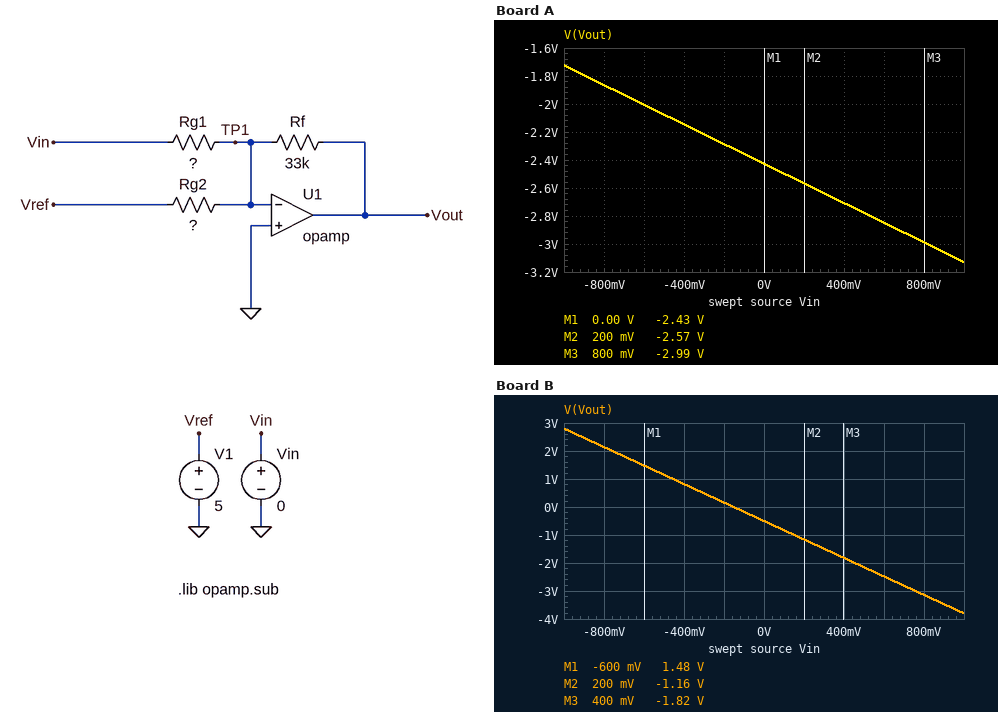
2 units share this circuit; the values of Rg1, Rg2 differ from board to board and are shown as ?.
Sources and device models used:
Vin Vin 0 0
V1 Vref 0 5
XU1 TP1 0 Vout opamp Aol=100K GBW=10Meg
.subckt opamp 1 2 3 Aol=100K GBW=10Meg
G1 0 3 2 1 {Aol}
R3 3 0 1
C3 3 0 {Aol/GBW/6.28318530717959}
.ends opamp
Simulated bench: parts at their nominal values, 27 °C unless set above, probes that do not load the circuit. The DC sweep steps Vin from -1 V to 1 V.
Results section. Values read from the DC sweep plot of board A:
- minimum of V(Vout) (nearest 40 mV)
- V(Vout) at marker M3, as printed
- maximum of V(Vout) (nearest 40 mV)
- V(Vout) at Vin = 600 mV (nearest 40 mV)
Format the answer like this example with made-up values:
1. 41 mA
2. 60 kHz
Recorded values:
1. -3.12 V
2. -2.99 V
3. -1.72 V
4. -2.84 V
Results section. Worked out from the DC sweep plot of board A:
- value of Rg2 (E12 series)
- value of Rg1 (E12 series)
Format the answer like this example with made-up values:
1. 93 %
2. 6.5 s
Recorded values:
1. 68 kΩ
2. 47 kΩ
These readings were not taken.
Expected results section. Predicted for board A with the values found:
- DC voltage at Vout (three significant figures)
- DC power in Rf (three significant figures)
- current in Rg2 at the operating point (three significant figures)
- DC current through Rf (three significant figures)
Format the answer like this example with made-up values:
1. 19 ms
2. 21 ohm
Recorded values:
1. -2.43 V
2. 178 µW
3. 73.5 µA
4. 73.5 µA
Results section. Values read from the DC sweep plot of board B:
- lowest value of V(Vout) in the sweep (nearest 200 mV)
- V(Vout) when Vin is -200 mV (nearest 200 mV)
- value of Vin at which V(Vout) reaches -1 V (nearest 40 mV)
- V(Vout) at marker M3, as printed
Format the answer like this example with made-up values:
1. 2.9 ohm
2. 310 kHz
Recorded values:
1. -3.8 V
2. 200 mV
3. 160 mV
4. -1.82 V
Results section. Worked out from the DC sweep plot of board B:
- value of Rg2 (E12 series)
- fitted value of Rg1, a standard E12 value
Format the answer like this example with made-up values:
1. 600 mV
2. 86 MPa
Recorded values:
1. 330 kΩ
2. 10 kΩ
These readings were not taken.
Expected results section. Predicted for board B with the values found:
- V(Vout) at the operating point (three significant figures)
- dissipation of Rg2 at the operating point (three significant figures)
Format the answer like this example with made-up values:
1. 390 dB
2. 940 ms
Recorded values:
1. -500 mV
2. 75.8 µW
